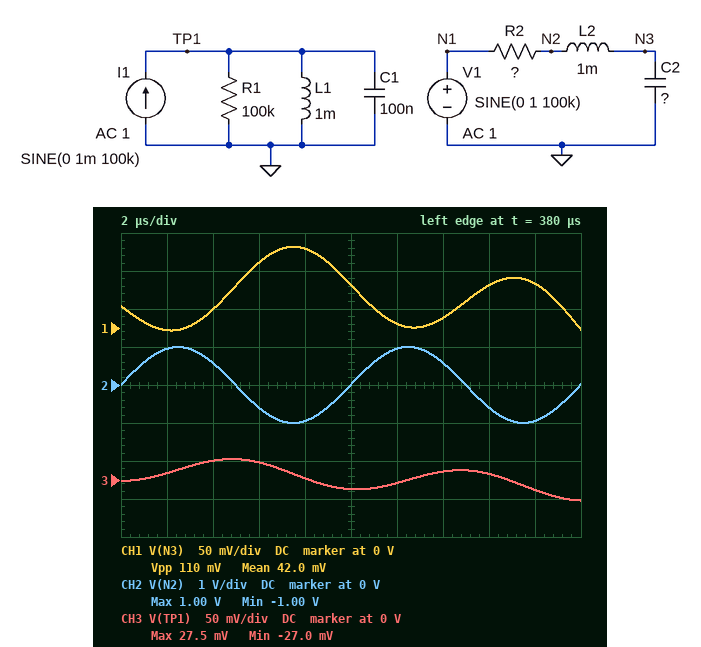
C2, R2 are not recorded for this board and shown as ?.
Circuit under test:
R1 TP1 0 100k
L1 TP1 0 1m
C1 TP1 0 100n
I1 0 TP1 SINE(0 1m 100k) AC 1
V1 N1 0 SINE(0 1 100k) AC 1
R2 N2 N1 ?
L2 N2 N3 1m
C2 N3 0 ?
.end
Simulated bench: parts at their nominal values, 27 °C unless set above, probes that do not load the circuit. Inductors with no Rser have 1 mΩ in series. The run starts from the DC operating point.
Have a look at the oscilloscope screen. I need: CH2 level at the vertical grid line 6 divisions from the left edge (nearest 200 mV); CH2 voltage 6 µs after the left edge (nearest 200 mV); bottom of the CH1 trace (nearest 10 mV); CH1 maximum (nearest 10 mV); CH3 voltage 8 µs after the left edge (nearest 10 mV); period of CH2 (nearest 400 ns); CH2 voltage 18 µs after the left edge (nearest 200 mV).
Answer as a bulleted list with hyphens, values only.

- 1.0 V
- -600 mV
- 0 V
- 110 mV
- 0 V
- 10.0 µs
- -1.0 V
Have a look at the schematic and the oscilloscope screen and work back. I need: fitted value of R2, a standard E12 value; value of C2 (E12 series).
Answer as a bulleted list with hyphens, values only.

- 6.8 Ω
- 56 nF
